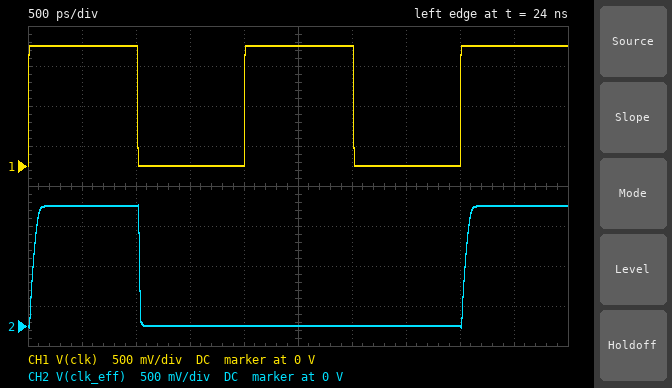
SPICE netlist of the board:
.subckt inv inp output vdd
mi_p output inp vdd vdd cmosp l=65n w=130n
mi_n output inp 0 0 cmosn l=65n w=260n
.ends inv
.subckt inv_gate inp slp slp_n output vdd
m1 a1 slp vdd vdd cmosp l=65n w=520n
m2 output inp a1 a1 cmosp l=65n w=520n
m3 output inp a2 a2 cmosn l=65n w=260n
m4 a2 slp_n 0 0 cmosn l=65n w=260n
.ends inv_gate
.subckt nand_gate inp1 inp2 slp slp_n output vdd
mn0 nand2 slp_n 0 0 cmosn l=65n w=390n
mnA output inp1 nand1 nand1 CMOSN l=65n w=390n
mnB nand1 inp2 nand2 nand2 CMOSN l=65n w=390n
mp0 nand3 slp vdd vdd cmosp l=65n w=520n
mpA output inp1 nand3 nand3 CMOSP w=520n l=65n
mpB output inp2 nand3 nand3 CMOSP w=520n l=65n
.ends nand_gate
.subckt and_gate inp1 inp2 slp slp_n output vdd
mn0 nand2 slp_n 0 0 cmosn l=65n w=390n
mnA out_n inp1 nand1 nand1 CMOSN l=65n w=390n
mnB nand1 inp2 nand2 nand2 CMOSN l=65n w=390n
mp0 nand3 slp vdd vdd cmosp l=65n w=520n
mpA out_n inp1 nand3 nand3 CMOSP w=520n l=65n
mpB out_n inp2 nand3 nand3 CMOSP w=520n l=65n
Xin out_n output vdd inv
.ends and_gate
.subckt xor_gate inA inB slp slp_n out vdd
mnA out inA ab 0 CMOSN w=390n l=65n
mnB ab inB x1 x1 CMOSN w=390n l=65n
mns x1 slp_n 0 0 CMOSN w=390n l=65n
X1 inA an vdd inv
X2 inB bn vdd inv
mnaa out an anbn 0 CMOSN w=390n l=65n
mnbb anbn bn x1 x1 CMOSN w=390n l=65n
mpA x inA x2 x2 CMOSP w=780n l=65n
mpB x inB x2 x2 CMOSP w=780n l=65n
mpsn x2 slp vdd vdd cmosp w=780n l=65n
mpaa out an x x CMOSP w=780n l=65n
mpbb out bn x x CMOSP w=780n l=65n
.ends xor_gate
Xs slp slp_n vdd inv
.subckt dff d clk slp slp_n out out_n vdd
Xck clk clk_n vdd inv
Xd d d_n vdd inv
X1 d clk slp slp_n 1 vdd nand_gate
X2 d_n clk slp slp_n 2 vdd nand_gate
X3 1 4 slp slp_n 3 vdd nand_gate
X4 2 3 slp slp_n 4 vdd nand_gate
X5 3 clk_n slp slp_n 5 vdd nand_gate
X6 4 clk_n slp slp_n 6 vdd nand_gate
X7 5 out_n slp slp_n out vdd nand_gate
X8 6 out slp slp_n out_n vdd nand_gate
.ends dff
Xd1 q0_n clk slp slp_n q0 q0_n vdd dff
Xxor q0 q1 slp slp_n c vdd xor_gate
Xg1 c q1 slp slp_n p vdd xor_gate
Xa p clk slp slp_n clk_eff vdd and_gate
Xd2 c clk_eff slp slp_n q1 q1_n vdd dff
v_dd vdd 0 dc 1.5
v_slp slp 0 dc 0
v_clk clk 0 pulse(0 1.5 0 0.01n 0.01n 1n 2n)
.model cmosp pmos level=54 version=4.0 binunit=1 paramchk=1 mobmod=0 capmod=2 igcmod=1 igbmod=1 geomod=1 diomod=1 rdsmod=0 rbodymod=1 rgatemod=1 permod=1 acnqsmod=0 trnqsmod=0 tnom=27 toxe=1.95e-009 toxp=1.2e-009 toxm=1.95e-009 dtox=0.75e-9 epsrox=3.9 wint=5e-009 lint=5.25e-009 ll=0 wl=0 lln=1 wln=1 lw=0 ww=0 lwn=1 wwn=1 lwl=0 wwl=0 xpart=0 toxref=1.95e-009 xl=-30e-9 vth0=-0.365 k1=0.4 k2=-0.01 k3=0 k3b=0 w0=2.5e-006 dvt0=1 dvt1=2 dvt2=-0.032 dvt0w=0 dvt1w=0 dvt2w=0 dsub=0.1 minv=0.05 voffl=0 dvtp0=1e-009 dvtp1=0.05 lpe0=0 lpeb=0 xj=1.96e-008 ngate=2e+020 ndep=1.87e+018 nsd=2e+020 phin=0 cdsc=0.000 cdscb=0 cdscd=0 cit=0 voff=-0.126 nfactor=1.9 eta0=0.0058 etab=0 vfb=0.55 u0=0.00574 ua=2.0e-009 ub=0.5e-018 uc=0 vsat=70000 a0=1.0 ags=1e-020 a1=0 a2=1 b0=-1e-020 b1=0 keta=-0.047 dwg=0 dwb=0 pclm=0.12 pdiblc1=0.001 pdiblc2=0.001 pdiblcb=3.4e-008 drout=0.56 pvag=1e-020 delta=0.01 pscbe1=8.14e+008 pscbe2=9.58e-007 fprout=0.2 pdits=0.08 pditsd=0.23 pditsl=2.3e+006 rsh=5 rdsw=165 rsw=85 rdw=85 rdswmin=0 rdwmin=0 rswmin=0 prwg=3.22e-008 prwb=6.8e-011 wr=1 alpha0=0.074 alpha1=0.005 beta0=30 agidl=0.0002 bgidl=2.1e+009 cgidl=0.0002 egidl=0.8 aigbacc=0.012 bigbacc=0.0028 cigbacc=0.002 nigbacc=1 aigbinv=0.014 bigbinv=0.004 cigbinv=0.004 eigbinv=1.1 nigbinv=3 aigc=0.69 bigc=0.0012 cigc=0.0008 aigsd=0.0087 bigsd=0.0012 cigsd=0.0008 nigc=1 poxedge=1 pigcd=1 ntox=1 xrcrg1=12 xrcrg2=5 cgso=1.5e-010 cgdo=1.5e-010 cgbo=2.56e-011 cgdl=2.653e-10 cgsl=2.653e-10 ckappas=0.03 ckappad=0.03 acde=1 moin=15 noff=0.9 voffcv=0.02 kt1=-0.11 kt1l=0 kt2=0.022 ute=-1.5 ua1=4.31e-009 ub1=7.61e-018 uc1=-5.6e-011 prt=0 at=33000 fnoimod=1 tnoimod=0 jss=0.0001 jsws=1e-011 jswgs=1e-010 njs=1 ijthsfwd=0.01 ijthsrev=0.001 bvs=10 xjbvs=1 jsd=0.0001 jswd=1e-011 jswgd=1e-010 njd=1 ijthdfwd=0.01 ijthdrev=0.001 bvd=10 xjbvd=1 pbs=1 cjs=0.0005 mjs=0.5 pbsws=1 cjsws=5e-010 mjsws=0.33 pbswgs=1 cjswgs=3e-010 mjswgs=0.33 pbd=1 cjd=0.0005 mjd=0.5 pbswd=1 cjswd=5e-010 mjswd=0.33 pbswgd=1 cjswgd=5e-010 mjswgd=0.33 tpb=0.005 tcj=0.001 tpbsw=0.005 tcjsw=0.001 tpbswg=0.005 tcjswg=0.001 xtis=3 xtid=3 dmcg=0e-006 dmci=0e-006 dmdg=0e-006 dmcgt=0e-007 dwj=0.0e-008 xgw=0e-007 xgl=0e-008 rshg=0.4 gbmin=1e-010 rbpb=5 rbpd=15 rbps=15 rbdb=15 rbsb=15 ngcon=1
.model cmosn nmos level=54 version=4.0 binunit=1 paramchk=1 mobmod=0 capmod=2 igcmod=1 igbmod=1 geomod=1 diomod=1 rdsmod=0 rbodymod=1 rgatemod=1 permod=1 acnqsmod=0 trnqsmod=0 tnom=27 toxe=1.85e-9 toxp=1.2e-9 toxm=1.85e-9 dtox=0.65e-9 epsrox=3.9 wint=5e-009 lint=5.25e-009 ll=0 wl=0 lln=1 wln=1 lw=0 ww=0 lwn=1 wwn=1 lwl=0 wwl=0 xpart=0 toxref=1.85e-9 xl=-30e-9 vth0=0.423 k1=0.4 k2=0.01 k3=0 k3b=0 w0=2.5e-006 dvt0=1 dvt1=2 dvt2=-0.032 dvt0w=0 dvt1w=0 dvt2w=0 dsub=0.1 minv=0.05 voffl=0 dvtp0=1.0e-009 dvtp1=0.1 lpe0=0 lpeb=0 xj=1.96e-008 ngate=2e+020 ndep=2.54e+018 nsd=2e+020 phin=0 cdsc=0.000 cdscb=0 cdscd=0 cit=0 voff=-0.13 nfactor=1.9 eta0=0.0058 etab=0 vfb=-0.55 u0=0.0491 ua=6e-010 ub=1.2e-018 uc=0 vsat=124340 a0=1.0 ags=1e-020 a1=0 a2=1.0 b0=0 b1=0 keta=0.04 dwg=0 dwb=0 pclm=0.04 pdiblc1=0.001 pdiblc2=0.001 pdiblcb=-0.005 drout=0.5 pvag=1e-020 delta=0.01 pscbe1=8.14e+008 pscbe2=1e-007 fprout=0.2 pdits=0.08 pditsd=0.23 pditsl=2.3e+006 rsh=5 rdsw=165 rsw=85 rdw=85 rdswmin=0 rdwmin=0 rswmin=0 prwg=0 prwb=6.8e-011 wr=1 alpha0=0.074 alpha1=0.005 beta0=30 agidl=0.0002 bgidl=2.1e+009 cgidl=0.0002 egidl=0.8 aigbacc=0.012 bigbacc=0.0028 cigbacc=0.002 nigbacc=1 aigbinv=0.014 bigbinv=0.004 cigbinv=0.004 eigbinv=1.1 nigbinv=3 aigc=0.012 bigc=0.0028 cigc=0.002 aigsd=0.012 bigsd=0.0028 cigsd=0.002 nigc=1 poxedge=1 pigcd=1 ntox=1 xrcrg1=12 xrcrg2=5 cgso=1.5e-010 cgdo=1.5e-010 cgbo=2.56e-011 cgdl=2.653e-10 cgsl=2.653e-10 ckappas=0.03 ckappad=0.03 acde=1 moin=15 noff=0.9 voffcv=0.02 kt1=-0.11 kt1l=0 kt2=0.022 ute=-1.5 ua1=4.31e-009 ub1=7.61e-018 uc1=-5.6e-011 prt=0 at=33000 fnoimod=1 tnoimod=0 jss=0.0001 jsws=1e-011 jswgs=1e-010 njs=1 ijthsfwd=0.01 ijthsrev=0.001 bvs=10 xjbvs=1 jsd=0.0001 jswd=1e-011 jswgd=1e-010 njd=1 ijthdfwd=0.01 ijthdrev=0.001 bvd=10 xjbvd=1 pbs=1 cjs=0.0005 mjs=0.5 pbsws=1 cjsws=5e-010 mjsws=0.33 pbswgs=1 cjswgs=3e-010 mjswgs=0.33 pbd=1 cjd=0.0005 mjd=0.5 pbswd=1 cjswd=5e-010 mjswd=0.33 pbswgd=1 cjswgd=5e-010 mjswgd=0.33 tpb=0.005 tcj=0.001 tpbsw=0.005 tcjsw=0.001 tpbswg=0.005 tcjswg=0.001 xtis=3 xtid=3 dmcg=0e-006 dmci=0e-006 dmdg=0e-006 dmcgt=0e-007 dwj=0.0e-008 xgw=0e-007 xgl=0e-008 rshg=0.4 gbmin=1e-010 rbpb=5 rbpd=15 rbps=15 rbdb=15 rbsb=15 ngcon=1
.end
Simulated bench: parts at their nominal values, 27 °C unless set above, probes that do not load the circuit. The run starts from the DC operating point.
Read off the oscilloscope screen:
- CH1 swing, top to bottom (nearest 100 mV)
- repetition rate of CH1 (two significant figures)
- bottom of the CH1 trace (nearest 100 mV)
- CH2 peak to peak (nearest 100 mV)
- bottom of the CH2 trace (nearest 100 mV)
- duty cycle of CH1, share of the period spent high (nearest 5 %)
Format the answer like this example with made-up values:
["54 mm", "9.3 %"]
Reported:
["1.5 V", "500 MHz", "0 V", "1.5 V", "0 V", "50 %"]
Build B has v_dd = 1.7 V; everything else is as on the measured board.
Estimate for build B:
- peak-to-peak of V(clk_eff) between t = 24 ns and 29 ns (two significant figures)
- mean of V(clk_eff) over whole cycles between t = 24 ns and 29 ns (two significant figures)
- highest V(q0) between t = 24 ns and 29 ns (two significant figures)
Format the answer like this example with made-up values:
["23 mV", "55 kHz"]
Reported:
["1.7 V", "420 mV", "1.8 V"]
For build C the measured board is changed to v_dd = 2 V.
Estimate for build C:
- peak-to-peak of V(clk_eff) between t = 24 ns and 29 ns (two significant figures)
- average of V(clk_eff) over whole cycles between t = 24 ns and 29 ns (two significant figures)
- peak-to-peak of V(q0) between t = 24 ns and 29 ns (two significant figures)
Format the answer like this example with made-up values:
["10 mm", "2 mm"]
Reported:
["2.0 V", "480 mV", "2.1 V"]
